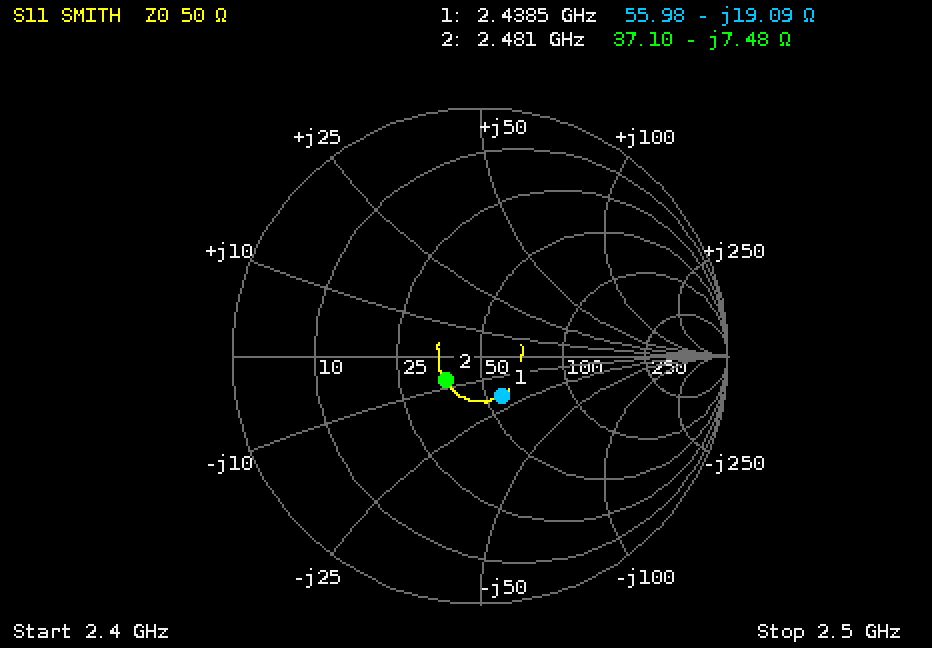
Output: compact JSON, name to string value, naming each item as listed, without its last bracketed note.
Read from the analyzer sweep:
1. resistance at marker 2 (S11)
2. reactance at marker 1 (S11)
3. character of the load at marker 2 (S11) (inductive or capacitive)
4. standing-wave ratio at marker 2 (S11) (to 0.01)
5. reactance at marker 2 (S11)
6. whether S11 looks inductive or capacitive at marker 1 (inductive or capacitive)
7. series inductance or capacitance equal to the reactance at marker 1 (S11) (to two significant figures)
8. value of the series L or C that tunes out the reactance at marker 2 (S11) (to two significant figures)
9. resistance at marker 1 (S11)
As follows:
{"resistance at marker 2": "37.10 Ω", "reactance at marker 1": "-19.09 Ω", "character of the load at marker 2 (S11)": "capacitive", "standing-wave ratio at marker 2 (S11)": "1.41", "reactance at marker 2": "-7.48 Ω", "whether S11 looks inductive or capacitive at marker 1": "capacitive", "series inductance or capacitance equal to the reactance at marker 1 (S11)": "3.4 pF", "value of the series L or C that tunes out the reactance at marker 2 (S11)": "480 pH", "resistance at marker 1": "55.98 Ω"}
